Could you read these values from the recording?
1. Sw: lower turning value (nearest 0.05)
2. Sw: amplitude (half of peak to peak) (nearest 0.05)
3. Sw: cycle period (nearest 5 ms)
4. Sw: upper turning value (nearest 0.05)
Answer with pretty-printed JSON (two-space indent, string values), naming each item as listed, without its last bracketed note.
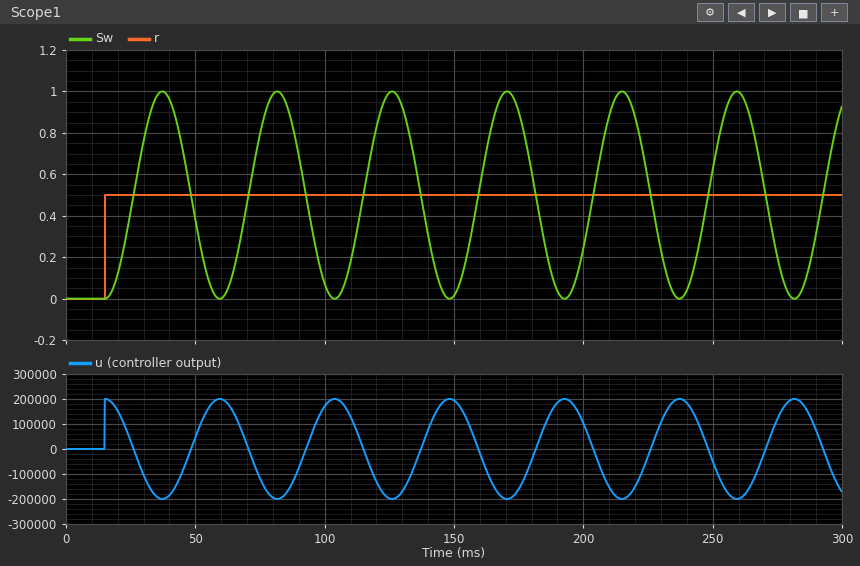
{
  "Sw: lower turning value": "0.00",
  "Sw: amplitude (half of peak to peak)": "0.50",
  "Sw: cycle period": "45 ms",
  "Sw: upper turning value": "1.00"
}
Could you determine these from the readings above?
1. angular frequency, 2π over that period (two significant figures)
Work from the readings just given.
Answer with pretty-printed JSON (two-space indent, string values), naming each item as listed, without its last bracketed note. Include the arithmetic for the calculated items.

{
  "angular frequency, 2π over that period": "2π / 45 = 0.14 rad/ms"
}
